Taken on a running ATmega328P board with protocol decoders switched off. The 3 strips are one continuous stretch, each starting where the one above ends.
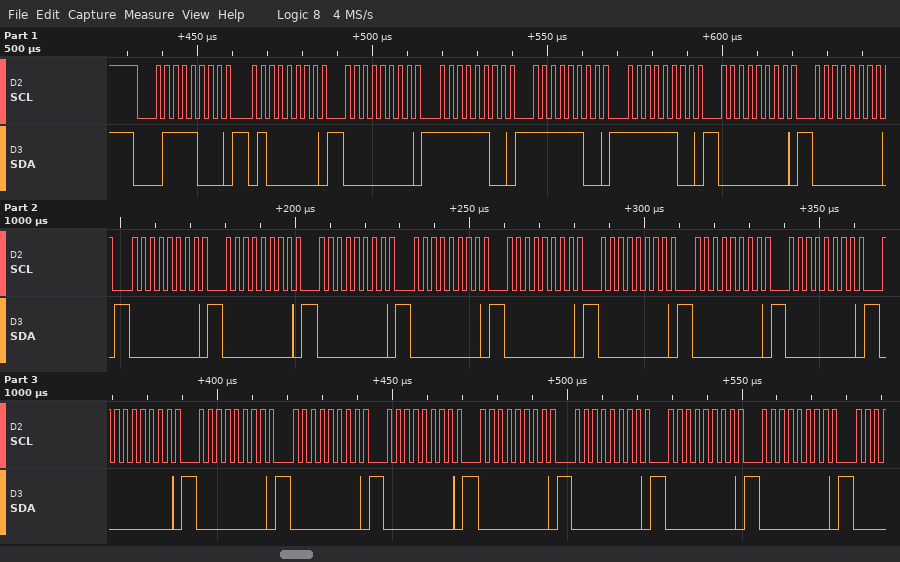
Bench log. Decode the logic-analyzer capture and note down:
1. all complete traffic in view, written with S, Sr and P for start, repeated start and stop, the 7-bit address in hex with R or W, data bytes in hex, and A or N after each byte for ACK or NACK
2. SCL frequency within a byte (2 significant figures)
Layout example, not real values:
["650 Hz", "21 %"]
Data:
["S 3CW A 40 A 00 A FC A FC A FC A 00 A 00 A 00 A 00 A 00 A 00 A 00 A 00 A 00 A 00 A 00 A 00 A 00 A 00 A 00 A 00 A 00 A 00 A", "400 kHz"]
